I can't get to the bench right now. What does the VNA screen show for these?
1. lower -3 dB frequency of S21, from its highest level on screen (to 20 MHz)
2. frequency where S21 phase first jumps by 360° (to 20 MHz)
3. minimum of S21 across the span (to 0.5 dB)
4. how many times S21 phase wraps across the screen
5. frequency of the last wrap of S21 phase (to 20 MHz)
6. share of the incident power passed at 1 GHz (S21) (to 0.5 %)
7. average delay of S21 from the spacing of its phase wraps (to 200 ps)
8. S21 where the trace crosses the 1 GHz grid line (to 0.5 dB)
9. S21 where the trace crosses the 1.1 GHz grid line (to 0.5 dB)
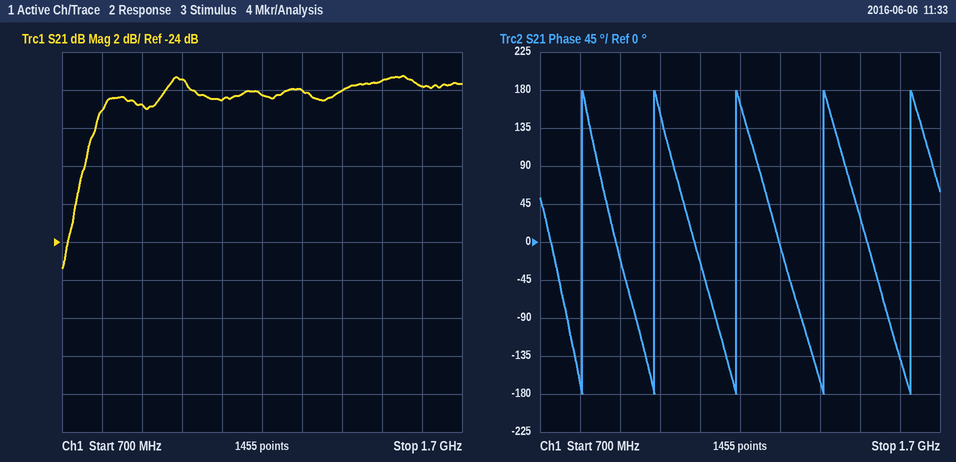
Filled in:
780 MHz
800 MHz
-25.5 dB
5
1.62 GHz
3.0 %
4.8 ns
-15.5 dB
-16.5 dB
